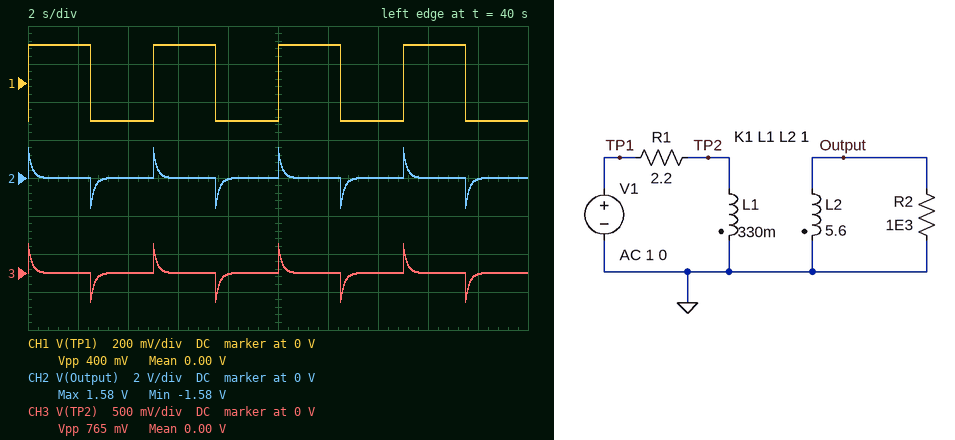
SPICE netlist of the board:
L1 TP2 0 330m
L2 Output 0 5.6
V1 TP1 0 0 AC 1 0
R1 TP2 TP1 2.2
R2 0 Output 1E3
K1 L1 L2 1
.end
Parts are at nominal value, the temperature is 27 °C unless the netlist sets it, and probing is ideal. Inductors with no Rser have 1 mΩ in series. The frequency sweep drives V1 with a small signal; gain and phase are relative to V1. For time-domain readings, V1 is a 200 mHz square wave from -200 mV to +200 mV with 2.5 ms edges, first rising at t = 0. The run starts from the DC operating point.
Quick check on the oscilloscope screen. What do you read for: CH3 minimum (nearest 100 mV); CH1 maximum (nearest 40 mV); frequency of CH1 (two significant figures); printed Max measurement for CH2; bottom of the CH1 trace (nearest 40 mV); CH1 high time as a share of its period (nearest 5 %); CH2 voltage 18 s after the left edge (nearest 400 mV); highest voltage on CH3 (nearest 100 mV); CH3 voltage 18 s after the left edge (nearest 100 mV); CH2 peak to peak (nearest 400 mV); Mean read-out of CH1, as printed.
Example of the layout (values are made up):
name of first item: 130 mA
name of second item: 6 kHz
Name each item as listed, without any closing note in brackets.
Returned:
CH3 minimum: -400 mV
CH1 maximum: 200 mV
frequency of CH1: 200 mHz
printed Max measurement for CH2: 1.58 V
bottom of the CH1 trace: -200 mV
CH1 high time as a share of its period: 50 %
CH2 voltage 18 s after the left edge: 0 V
highest voltage on CH3: 400 mV
CH3 voltage 18 s after the left edge: 0 V
CH2 peak to peak: 3.2 V
Mean read-out of CH1, as printed: 0.00 V
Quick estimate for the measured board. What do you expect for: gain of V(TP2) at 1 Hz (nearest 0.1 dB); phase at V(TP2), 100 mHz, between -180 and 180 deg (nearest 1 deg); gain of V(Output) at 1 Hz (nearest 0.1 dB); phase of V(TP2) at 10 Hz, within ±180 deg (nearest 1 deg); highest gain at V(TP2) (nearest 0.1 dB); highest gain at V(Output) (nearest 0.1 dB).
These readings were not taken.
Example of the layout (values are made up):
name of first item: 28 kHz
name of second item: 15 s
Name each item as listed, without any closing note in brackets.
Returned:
gain of V(TP2) at 1 Hz: -3.4 dB
phase at V(TP2), 100 mHz, between -180 and 180 deg: 84 deg
gain of V(Output) at 1 Hz: 8.9 dB
phase of V(TP2) at 10 Hz, within ±180 deg: 6 deg
highest gain at V(TP2): -0.3 dB
highest gain at V(Output): 12.0 dB
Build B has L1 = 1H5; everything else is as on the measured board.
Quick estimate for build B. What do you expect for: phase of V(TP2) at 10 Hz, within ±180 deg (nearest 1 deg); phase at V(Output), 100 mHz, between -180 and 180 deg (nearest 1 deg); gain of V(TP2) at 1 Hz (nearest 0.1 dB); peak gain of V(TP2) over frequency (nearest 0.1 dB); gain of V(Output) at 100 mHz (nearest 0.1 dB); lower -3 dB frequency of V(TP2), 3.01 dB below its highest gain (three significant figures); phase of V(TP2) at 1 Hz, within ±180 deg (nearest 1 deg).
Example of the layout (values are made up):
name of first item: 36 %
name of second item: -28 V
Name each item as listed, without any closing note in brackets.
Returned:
phase of V(TP2) at 10 Hz, within ±180 deg: 1 deg
phase at V(Output), 100 mHz, between -180 and 180 deg: 67 deg
gain of V(TP2) at 1 Hz: -0.3 dB
peak gain of V(TP2) over frequency: -0.1 dB
gain of V(Output) at 100 mHz: -2.4 dB
lower -3 dB frequency of V(TP2), 3.01 dB below its highest gain: 232 mHz
phase of V(TP2) at 1 Hz, within ±180 deg: 13 deg
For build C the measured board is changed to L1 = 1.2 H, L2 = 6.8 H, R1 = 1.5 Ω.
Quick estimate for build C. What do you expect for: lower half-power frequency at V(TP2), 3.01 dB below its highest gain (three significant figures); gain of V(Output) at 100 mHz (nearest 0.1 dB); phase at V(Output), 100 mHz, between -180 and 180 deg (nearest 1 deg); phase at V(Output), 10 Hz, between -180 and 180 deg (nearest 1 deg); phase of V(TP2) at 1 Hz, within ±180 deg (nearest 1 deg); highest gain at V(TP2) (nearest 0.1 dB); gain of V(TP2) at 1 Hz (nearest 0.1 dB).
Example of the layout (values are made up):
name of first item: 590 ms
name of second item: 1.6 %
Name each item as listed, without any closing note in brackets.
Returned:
lower half-power frequency at V(TP2), 3.01 dB below its highest gain: 197 mHz
gain of V(Output) at 100 mHz: 0.6 dB
phase at V(Output), 100 mHz, between -180 and 180 deg: 63 deg
phase at V(Output), 10 Hz, between -180 and 180 deg: 1 deg
phase of V(TP2) at 1 Hz, within ±180 deg: 11 deg
highest gain at V(TP2): -0.1 dB
gain of V(TP2) at 1 Hz: -0.2 dB
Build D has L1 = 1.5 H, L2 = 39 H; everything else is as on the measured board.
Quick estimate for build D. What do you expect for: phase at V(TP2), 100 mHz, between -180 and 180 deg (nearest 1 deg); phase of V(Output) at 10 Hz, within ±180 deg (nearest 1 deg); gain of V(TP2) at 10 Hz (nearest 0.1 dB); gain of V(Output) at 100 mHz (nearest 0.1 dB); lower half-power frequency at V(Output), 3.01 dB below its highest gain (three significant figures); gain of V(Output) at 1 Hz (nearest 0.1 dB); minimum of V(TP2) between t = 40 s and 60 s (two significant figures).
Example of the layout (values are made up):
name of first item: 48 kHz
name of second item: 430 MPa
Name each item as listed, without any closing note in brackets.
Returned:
phase at V(TP2), 100 mHz, between -180 and 180 deg: 66 deg
phase of V(Output) at 10 Hz, within ±180 deg: 1 deg
gain of V(TP2) at 10 Hz: -0.5 dB
gain of V(Output) at 100 mHz: 6.0 dB
lower half-power frequency at V(Output), 3.01 dB below its highest gain: 221 mHz
gain of V(Output) at 1 Hz: 13.5 dB
minimum of V(TP2) between t = 40 s and 60 s: -370 mV
